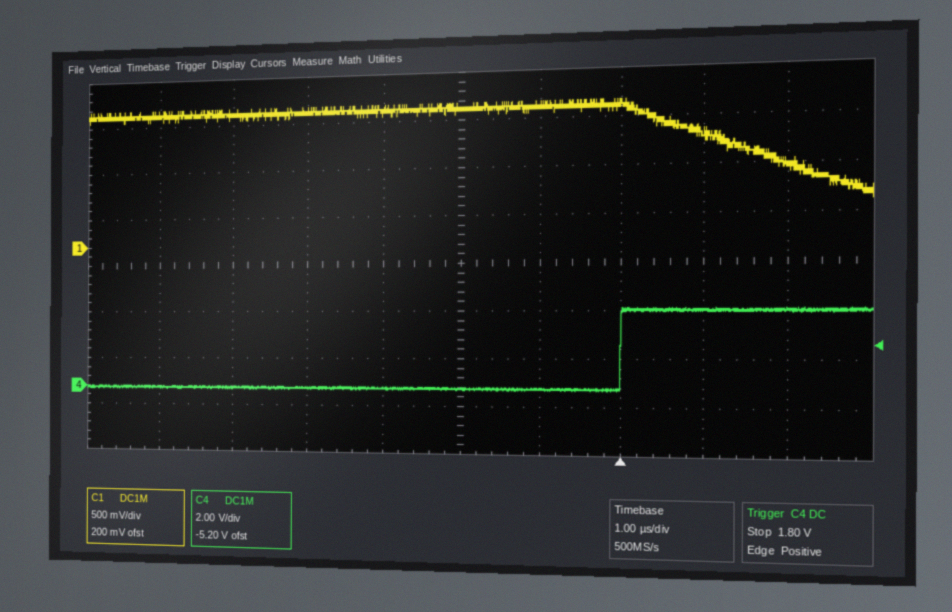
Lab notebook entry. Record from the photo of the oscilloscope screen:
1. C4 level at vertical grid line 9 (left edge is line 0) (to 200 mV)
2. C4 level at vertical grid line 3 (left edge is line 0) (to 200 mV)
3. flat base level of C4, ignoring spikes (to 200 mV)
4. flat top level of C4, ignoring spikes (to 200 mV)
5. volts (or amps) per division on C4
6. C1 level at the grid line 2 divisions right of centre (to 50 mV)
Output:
3.2 V
0.0 V
0.0 V
3.2 V
2 V
1.45 V
